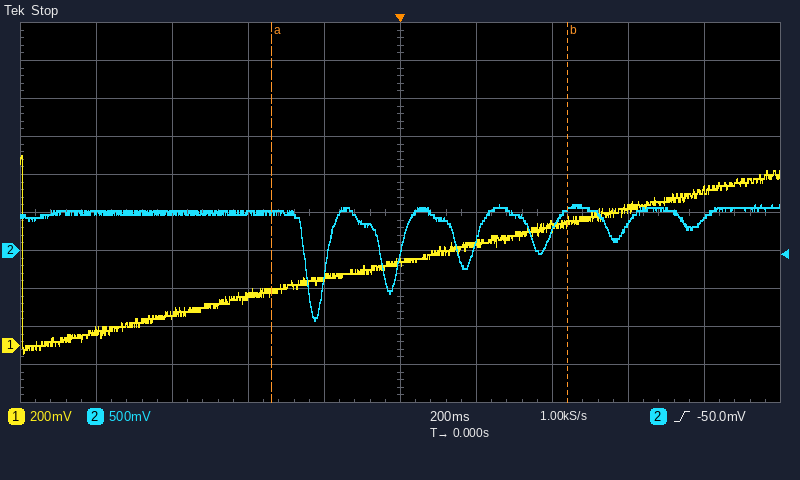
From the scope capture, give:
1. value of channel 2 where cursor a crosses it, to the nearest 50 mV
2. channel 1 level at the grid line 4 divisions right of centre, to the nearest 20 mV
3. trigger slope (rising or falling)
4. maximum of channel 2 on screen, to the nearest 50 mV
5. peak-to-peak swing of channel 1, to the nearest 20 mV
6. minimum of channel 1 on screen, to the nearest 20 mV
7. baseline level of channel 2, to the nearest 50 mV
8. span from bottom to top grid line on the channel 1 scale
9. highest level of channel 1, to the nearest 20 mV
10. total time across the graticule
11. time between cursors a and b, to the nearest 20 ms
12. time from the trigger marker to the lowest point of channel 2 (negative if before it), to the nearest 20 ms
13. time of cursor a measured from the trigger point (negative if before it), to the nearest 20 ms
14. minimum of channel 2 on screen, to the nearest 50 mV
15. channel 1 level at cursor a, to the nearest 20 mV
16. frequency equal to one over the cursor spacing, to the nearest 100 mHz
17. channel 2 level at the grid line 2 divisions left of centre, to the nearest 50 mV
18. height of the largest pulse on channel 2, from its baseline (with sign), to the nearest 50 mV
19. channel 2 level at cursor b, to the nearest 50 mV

500 mV
820 mV
rising
600 mV
1.04 V
-40 mV
500 mV
2 V
1.00 V
2 s
780 ms
-220 ms
-340 ms
-900 mV
280 mV
1.3 Hz
500 mV
-1.40 V
550 mV
